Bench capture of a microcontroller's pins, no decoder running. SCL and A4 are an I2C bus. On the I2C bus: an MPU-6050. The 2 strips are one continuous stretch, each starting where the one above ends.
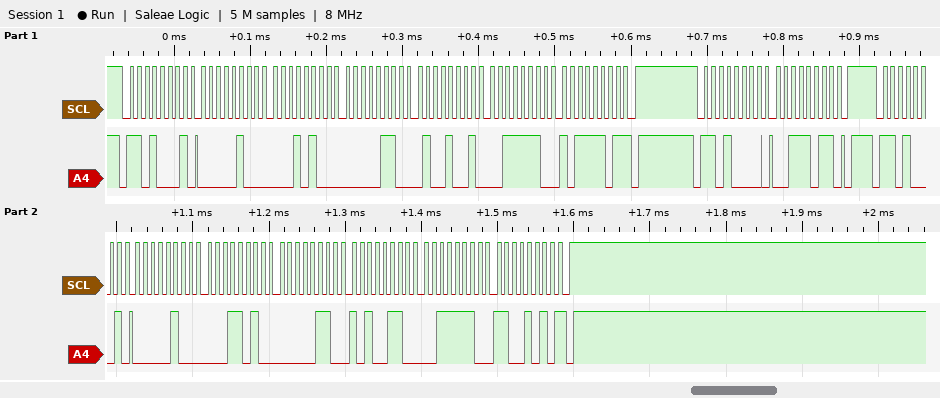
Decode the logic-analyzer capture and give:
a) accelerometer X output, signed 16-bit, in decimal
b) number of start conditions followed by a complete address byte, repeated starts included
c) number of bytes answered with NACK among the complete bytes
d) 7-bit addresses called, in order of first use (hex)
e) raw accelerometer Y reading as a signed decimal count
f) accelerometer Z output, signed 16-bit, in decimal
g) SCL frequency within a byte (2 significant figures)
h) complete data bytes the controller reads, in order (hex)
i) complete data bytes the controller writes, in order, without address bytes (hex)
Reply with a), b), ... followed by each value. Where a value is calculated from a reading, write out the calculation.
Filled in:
a) 0x041A = 1050
b) 3
c) 2
d) 0x68
e) 0x06A6 = 1702
f) 0x3ECA = 16074
g) 100 kHz
h) 04 14 06 49 3E BD 04 1A 06 A6 3E CA
i) 3B
